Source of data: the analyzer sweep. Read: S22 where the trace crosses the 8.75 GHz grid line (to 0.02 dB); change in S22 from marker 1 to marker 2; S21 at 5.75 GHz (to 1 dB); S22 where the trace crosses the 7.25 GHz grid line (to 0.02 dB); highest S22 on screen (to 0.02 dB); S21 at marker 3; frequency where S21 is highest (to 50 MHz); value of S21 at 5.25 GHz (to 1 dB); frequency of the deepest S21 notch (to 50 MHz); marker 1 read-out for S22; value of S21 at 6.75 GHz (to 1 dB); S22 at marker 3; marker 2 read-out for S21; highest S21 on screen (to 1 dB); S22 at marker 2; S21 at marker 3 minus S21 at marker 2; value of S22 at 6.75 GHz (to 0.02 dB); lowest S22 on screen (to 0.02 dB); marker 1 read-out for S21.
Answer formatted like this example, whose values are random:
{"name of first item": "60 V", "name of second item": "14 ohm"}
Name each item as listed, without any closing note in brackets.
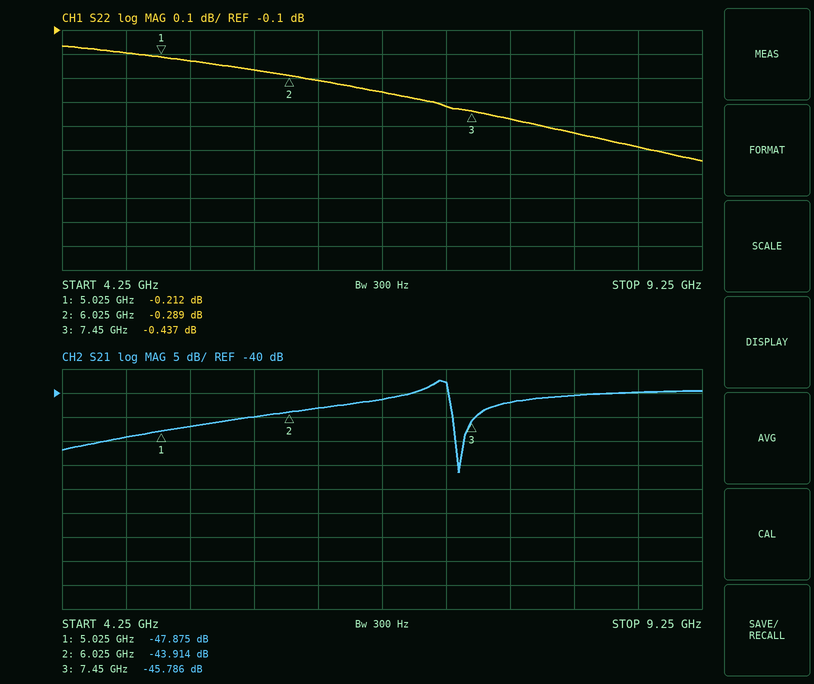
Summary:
{"S22 where the trace crosses the 8.75 GHz grid line": "-0.58 dB", "change in S22 from marker 1 to marker 2": "-0.077 dB", "S21 at 5.75 GHz": "-45 dB", "S22 where the trace crosses the 7.25 GHz grid line": "-0.42 dB", "highest S22 on screen": "-0.16 dB", "S21 at marker 3": "-45.786 dB", "frequency where S21 is highest": "7.20 GHz", "value of S21 at 5.25 GHz": "-47 dB", "frequency of the deepest S21 notch": "7.35 GHz", "marker 1 read-out for S22": "-0.212 dB", "value of S21 at 6.75 GHz": "-41 dB", "S22 at marker 3": "-0.437 dB", "marker 2 read-out for S21": "-43.914 dB", "highest S21 on screen": "-37 dB", "S22 at marker 2": "-0.289 dB", "S21 at marker 3 minus S21 at marker 2": "-1.872 dB", "value of S22 at 6.75 GHz": "-0.36 dB", "lowest S22 on screen": "-0.64 dB", "marker 1 read-out for S21": "-47.875 dB"}
